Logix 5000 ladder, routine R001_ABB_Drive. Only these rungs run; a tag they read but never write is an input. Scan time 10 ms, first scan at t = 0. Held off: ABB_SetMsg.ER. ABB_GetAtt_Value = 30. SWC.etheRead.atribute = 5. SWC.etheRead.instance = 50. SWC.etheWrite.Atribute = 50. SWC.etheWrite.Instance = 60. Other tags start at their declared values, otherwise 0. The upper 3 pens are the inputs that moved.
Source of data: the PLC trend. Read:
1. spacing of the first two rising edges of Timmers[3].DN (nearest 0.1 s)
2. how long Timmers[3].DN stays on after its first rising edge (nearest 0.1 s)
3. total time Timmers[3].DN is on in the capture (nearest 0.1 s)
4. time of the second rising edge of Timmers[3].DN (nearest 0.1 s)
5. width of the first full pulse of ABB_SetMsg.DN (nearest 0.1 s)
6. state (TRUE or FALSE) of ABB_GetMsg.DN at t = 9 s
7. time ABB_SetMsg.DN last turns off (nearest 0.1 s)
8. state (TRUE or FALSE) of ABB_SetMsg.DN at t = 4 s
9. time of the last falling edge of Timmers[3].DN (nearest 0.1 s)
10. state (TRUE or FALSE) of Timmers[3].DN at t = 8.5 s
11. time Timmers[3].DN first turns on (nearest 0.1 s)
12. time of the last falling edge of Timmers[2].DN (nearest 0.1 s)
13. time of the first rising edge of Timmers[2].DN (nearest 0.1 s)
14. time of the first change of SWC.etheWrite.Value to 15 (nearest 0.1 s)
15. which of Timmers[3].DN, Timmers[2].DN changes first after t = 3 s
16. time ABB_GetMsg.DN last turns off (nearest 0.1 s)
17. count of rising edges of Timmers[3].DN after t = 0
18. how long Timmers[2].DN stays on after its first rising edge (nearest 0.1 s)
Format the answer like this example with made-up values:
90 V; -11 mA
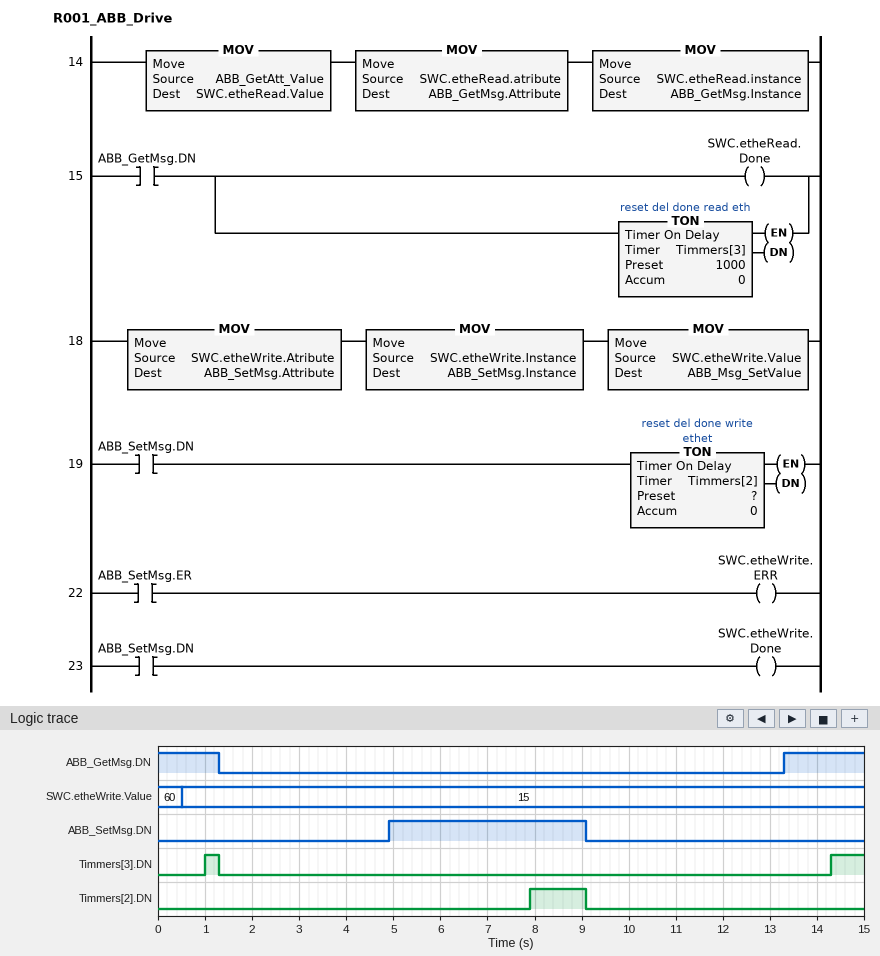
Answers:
13.3 s; 0.3 s; 1.0 s; 14.3 s; 4.2 s; FALSE; 9.1 s; FALSE; 1.3 s; FALSE; 1.0 s; 9.1 s; 7.9 s; 0.5 s; Timmers[2].DN; 1.3 s; 2; 1.2 s
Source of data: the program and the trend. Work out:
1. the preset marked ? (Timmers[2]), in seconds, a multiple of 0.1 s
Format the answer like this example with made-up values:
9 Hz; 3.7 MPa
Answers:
3.0 s
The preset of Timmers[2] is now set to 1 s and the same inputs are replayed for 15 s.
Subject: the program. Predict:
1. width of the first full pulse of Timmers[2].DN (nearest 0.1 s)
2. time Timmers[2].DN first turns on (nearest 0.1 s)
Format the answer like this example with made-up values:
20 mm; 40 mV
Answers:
3.2 s; 5.9 s
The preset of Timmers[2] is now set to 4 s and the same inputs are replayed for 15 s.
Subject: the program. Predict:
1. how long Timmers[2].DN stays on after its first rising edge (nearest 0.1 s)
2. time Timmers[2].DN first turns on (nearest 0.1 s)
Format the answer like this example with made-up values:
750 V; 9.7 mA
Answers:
0.2 s; 8.9 s
